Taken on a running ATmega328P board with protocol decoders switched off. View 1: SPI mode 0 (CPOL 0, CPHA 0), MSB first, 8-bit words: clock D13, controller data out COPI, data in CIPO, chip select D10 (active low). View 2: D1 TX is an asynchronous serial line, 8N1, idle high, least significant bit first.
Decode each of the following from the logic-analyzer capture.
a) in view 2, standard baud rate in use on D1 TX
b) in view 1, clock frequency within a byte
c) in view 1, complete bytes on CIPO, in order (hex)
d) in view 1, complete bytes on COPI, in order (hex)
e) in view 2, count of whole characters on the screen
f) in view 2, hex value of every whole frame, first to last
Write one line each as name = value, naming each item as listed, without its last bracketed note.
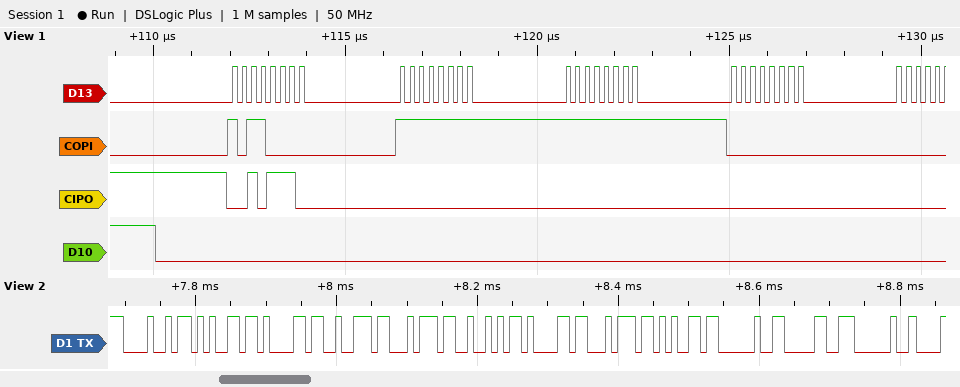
in view 2, standard baud rate in use on D1 TX = 115200 baud
in view 1, clock frequency within a byte = 4 MHz
in view 1, complete bytes on CIPO, in order = 0x2E 0x00 0x00 0x00
in view 1, complete bytes on COPI, in order = 0xB0 0xFF 0xFF 0x00
in view 2, count of whole characters on the screen = 12
in view 2, hex value of every whole frame, first to last = 0x48 0x65 0x61 0x72 0x74 0x52 0x61 0x74 0x65 0x20 0x30 0x20
